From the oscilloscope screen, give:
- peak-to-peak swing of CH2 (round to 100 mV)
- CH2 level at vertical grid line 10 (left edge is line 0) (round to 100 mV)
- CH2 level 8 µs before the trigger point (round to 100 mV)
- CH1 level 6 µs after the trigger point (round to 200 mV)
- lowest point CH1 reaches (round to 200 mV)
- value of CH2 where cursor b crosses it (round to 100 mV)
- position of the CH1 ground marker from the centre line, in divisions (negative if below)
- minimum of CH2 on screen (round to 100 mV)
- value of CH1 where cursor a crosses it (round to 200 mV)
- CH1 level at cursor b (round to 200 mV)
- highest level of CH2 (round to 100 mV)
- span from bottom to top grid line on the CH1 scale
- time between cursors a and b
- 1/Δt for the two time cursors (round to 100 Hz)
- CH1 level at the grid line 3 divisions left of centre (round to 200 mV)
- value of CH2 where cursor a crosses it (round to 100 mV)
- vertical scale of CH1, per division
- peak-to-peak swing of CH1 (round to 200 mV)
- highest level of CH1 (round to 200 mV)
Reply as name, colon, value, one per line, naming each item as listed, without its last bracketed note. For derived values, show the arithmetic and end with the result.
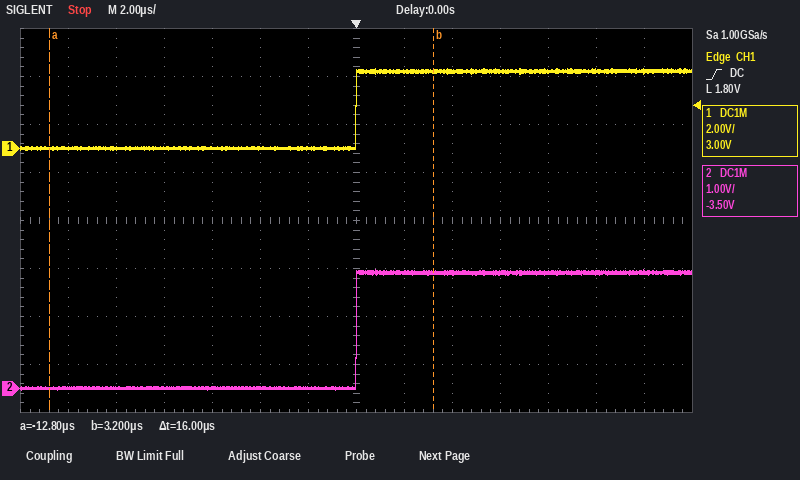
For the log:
peak-to-peak swing of CH2: 2.5 V − (0.0 V) = 2.5 V
CH2 level at vertical grid line 10 (left edge is line 0): 2.4 V
CH2 level 8 µs before the trigger point: 0.0 V
CH1 level 6 µs after the trigger point: 3.2 V
lowest point CH1 reaches: 0.0 V
value of CH2 where cursor b crosses it: 2.4 V
position of the CH1 ground marker from the centre line, in divisions: +1.5 div
minimum of CH2 on screen: 0.0 V
value of CH1 where cursor a crosses it: 0.0 V
CH1 level at cursor b: 3.2 V
highest level of CH2: 2.5 V
span from bottom to top grid line on the CH1 scale: 16 V
time between cursors a and b: 16 µs
1/Δt for the two time cursors: 1 / 16 µs ≈ 62.5 kHz
CH1 level at the grid line 3 divisions left of centre: 0.0 V
value of CH2 where cursor a crosses it: 0.0 V
vertical scale of CH1, per division: 2 V
peak-to-peak swing of CH1: 3.4 V − (0.0 V) = 3.4 V
highest level of CH1: 3.4 V
